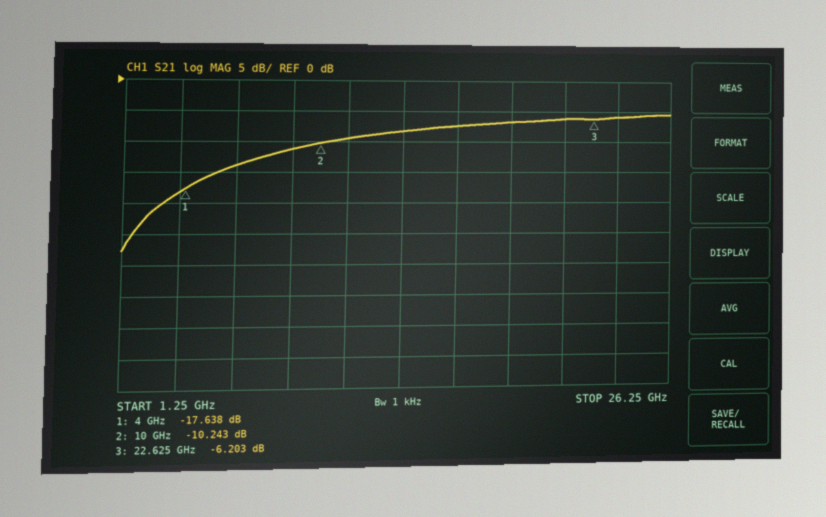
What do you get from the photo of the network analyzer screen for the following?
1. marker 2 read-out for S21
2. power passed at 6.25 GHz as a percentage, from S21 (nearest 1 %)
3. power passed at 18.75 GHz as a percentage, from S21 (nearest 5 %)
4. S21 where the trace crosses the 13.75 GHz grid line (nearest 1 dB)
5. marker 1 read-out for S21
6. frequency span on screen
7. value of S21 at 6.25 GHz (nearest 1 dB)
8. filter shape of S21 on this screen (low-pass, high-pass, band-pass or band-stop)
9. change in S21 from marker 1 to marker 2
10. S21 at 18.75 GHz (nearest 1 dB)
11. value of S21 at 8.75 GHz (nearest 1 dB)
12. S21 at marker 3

-10.243 dB
4 %
20 %
-8 dB
-17.638 dB
25 GHz
-14 dB
high-pass
7.395 dB
-7 dB
-11 dB
-6.203 dB
